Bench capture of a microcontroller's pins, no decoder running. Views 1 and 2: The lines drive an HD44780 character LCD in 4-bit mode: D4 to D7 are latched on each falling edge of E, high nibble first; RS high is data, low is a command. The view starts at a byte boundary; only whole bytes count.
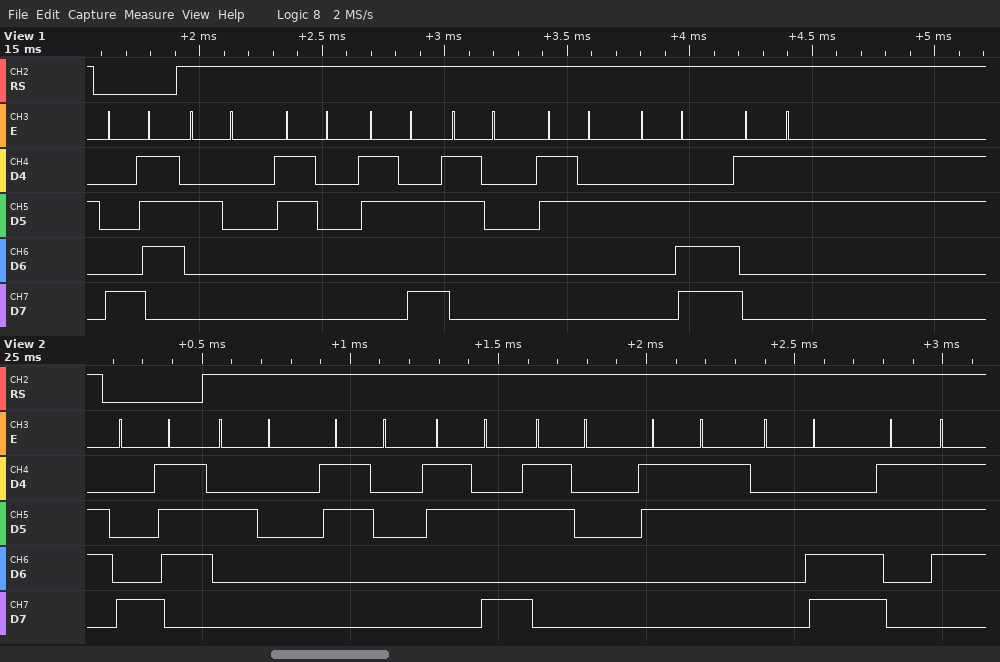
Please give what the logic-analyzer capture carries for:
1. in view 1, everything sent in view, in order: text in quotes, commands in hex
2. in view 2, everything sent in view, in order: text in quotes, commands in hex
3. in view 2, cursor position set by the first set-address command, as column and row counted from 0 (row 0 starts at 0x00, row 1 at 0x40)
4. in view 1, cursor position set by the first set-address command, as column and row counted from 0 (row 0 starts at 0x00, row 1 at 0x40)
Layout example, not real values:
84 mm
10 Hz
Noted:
0x87 " 0:02.3"
0x87 " 0:03.7"
column 7, row 0
column 7, row 0
